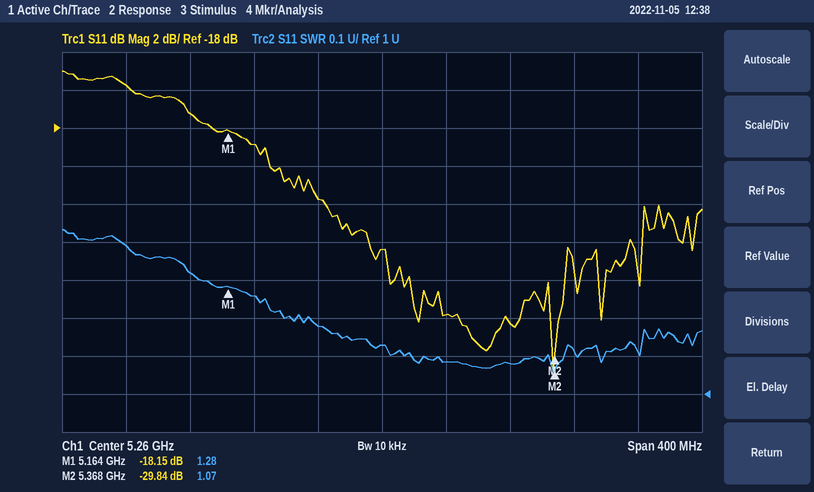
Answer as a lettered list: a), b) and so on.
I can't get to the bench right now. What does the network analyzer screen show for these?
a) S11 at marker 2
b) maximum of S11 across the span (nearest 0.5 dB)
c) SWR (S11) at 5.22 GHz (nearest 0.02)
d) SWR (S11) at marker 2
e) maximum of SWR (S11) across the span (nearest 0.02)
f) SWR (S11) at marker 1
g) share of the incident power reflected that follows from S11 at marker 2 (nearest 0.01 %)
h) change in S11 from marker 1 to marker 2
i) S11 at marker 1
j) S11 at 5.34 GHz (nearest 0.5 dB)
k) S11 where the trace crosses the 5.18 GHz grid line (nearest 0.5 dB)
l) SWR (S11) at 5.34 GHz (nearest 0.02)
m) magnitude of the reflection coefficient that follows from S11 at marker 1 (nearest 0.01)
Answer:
a) -29.84 dB
b) -15.0 dB
c) 1.18
d) 1.07
e) 1.44
f) 1.28
g) 0.10 %
h) -11.69 dB
i) -18.15 dB
j) -28.5 dB
k) -19.0 dB
l) 1.08
m) 0.12
